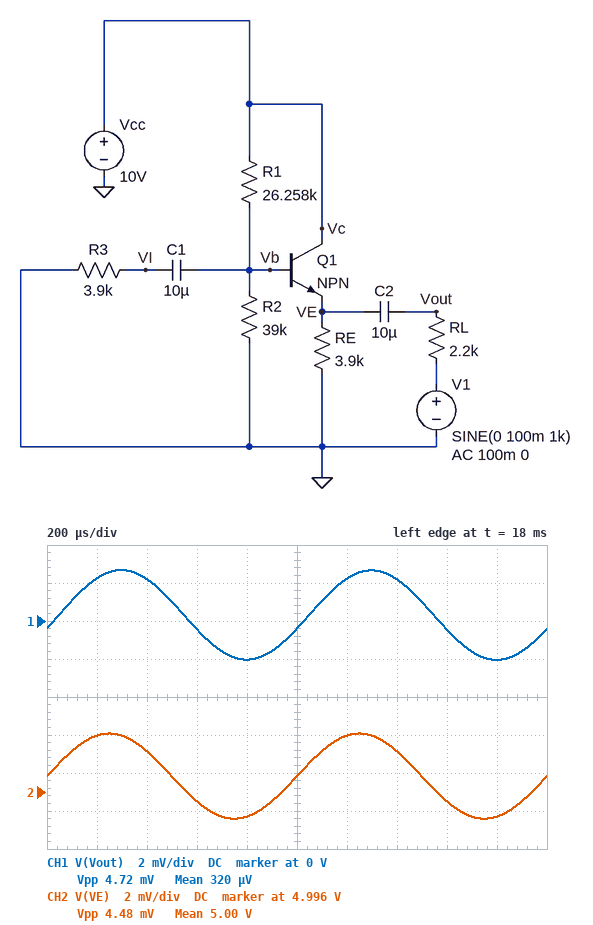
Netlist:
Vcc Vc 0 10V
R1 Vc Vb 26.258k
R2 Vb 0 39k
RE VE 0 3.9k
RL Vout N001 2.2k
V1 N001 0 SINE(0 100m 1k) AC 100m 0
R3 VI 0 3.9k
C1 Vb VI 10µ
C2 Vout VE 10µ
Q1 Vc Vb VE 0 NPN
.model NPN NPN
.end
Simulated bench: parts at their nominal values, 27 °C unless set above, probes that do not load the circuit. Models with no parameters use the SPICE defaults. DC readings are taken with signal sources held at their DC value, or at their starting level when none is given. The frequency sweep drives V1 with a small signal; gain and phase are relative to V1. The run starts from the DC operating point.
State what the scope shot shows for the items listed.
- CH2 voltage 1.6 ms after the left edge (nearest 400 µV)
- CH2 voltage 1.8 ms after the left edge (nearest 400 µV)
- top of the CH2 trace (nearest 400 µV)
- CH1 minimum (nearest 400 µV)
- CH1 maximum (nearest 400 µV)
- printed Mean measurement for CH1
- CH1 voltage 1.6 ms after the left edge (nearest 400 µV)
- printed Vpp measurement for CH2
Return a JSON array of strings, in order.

["4.9956 V", "4.9948 V", "4.9992 V", "-2.0 mV", "2.8 mV", "320 µV", "-400 µV", "4.48 mV"]
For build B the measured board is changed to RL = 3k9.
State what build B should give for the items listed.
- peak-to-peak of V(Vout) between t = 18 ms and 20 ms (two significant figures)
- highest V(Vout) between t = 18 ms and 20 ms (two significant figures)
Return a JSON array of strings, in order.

["2.7 mV", "1.6 mV"]
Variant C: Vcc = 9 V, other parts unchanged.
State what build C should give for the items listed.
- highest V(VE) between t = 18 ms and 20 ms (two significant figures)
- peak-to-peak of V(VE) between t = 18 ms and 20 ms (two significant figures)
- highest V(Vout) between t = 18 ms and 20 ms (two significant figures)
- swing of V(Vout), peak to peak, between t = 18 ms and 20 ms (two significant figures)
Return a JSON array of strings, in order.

["4.4 V", "4.7 mV", "2.8 mV", "4.9 mV"]
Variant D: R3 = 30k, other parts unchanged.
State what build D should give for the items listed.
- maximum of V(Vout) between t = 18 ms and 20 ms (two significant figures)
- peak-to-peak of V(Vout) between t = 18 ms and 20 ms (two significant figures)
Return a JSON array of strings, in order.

["5.5 mV", "10 mV"]
